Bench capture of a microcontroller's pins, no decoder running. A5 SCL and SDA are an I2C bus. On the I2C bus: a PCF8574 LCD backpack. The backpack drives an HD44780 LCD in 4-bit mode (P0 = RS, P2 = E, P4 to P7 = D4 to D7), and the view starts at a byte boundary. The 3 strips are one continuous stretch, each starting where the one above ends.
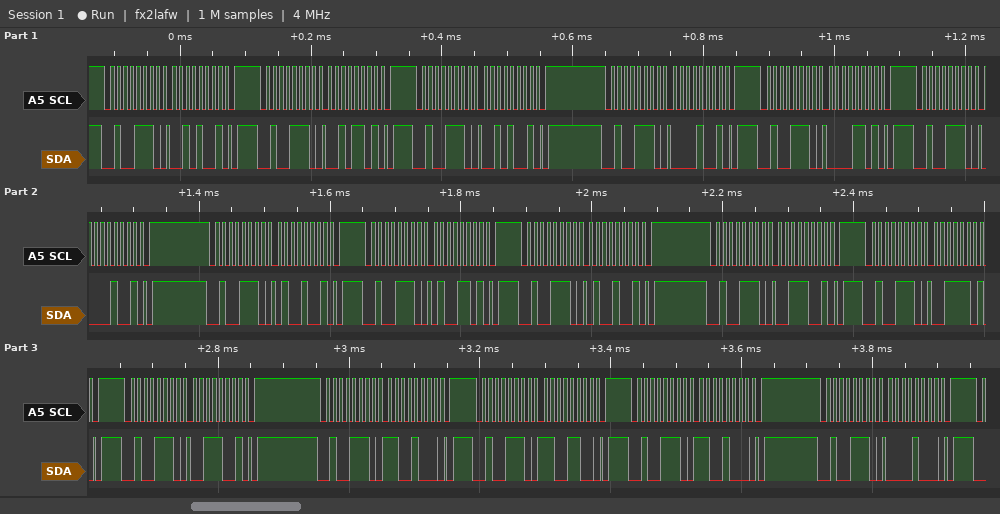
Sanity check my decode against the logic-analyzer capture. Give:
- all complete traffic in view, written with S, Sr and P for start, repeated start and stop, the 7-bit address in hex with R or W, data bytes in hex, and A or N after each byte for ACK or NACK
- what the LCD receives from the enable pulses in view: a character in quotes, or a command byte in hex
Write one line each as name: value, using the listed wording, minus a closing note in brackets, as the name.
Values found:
all complete traffic in view, written with S, Sr and P for start, repeated start and stop, the 7-bit address in hex with R or W, data bytes in hex, and A or N after each byte for ACK or NACK: S 27W A 29 A P S 27W A 2D A P S 27W A 29 A P S 27W A 09 A P S 27W A 0D A P S 27W A 09 A P S 27W A 49 A P S 27W A 4D A P S 27W A 49 A P S 27W A 39 A P S 27W A 3D A P S 27W A 39 A P S 27W A C8 A P S 27W A CC A P S 27W A C8 A P S 27W A 08 A P
what the LCD receives from the enable pulses in view: a character in quotes, or a command byte in hex: ' ' 'C'
